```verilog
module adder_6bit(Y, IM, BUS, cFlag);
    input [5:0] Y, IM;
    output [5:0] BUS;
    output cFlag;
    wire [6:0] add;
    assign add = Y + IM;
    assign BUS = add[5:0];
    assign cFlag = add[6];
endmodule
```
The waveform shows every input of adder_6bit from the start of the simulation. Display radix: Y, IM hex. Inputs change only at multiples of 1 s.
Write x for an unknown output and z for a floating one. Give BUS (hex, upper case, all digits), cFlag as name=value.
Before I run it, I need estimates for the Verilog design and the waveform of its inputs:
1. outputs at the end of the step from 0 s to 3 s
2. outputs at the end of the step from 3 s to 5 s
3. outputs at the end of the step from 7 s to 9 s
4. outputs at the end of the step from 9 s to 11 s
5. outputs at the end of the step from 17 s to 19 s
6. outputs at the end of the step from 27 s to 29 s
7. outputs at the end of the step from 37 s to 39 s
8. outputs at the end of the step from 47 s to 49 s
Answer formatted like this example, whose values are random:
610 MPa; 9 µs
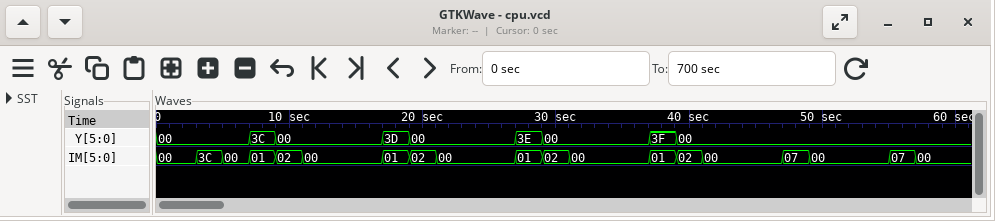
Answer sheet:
BUS=00, cFlag=0; BUS=3C, cFlag=0; BUS=3D, cFlag=0; BUS=02, cFlag=0; BUS=3E, cFlag=0; BUS=3F, cFlag=0; BUS=00, cFlag=1; BUS=07, cFlag=0
